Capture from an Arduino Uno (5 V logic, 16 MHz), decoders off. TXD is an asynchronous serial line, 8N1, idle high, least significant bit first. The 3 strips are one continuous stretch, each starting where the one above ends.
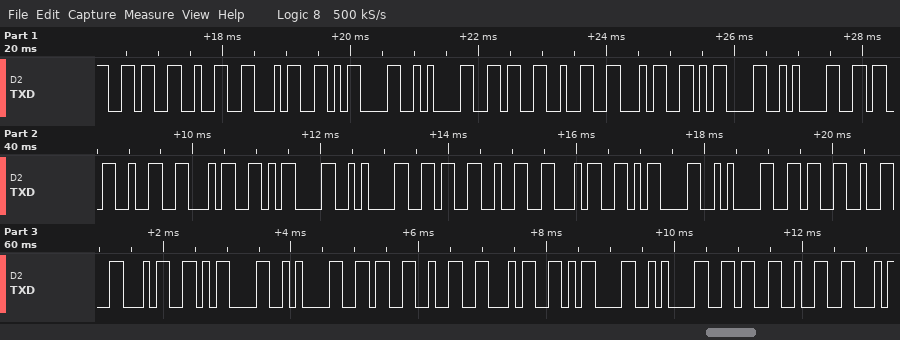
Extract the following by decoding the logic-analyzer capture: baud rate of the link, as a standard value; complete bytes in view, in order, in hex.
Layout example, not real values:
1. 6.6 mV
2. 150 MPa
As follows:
1. 9600 baud
2. 36 32 34 0D 0A 36 32 34 0D 0A 36 32 34 0D 0A 36 32 34 0D 0A 36 32 34 0D 0A 36 32 34 0D 0A 36 32
